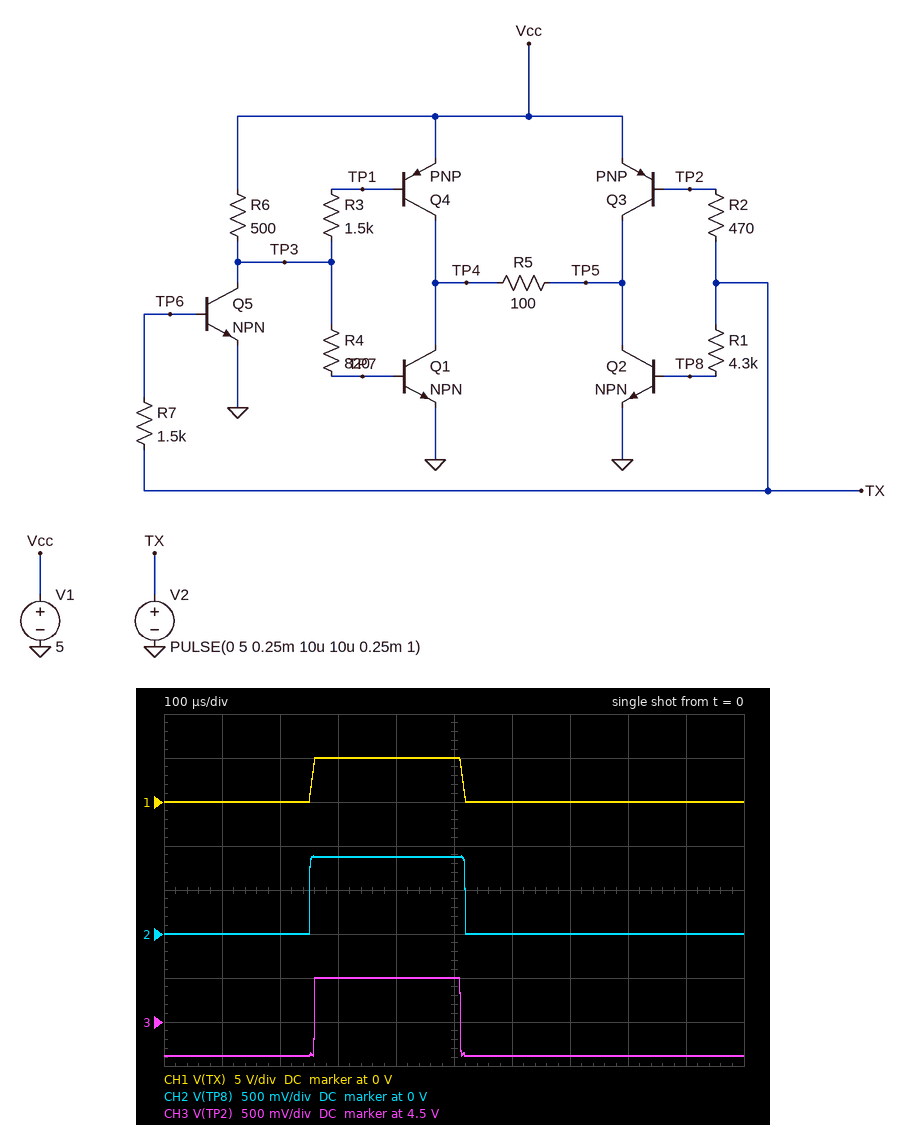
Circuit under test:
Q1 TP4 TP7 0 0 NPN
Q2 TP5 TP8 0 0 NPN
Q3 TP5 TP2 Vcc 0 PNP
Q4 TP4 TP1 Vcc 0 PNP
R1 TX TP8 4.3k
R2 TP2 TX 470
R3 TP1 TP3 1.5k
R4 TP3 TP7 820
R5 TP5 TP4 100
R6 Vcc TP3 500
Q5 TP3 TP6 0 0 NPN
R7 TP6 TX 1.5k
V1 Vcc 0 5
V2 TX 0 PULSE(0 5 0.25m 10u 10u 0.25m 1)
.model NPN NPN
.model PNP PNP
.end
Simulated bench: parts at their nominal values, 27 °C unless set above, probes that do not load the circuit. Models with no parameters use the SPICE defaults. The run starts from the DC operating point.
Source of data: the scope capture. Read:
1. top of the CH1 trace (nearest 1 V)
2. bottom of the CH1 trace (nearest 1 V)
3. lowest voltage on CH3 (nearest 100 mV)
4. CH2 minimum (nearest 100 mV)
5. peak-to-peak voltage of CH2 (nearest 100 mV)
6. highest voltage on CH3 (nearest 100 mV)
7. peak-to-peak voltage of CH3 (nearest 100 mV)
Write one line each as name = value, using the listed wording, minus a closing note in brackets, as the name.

top of the CH1 trace = 5 V
bottom of the CH1 trace = 0 V
lowest voltage on CH3 = 4.1 V
CH2 minimum = 0 V
peak-to-peak voltage of CH2 = 900 mV
highest voltage on CH3 = 5.0 V
peak-to-peak voltage of CH3 = 900 mV
